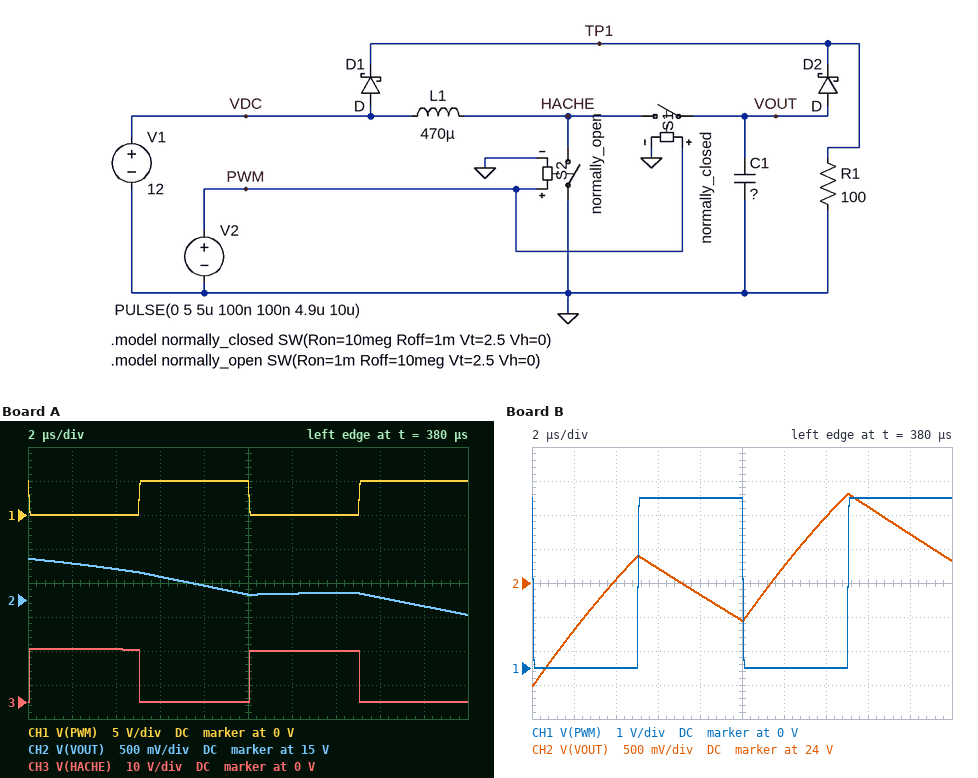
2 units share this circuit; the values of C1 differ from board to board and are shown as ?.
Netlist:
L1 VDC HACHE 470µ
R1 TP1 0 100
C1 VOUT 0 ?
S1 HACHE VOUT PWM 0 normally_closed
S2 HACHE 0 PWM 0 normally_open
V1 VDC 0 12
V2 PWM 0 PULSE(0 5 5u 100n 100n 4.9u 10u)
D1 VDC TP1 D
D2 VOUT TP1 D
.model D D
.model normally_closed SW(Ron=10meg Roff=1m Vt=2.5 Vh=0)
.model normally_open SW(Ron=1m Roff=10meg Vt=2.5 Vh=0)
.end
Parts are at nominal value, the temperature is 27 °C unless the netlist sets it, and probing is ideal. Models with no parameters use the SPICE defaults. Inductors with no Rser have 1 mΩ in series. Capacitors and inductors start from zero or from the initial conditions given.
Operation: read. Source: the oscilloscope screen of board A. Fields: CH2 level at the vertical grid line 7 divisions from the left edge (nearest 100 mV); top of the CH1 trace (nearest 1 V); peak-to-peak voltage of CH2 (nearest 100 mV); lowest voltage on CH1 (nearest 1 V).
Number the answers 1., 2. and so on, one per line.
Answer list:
1. 15.1 V
2. 5 V
3. 800 mV
4. 0 V
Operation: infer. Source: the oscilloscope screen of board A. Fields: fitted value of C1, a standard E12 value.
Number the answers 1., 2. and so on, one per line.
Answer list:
1. 2.2 µF
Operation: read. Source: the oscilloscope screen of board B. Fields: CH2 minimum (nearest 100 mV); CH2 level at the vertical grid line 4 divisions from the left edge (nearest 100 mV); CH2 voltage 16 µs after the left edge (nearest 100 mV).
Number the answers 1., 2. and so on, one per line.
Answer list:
1. 22.5 V
2. 23.8 V
3. 25.1 V
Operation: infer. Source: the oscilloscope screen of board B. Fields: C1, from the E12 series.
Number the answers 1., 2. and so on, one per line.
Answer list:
1. 1.2 µF
